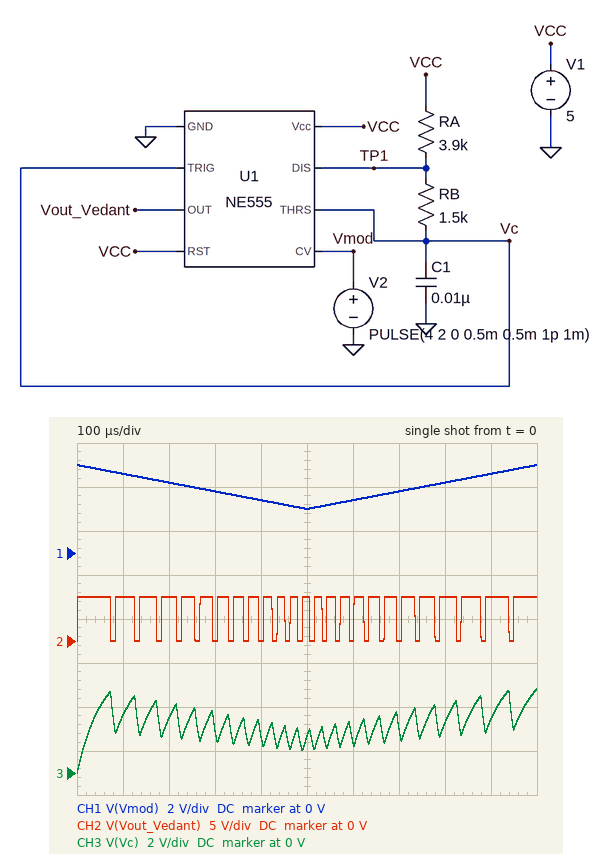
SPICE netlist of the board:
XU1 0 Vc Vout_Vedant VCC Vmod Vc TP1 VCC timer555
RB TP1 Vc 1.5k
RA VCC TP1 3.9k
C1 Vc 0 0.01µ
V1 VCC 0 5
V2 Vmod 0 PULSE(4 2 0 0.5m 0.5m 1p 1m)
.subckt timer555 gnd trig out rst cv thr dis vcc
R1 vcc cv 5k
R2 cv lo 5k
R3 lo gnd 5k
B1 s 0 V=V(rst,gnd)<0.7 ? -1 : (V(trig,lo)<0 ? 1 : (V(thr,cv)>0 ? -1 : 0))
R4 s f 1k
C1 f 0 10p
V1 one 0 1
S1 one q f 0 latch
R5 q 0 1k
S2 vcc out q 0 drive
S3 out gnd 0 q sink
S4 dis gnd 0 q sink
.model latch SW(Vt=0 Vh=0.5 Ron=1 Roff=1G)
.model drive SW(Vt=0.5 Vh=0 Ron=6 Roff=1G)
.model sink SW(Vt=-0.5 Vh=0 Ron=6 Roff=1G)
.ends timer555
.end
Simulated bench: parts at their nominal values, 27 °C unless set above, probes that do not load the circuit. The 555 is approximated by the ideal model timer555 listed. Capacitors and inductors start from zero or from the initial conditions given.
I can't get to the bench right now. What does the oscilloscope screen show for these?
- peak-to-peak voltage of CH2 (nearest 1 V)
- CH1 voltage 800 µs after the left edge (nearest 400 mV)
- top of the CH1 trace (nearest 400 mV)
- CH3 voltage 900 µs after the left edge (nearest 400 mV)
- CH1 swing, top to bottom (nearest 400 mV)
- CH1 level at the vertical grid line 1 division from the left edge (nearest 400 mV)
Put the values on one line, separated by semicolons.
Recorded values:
5 V; 3.2 V; 4.0 V; 2.4 V; 2.0 V; 3.6 V
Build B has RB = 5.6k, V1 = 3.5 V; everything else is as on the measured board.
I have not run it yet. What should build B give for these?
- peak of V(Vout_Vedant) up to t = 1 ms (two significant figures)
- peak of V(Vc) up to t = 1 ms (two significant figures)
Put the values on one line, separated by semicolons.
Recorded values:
3.5 V; 3.4 V
